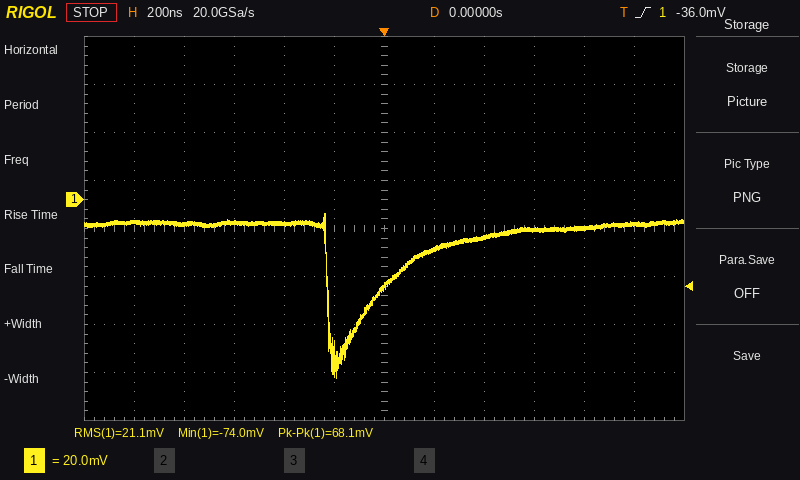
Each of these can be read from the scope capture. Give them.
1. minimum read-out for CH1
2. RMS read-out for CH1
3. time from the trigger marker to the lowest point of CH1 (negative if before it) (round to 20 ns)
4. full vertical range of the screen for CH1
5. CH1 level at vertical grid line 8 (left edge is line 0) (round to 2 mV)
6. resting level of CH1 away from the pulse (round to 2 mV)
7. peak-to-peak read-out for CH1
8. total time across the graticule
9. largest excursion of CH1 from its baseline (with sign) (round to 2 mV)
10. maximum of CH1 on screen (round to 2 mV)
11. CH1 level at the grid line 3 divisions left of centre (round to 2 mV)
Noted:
-74.0 mV
21.1 mV
-200 ns
160 mV
-16 mV
-10 mV
68.1 mV
2.4 µs
-64 mV
-6 mV
-10 mV
